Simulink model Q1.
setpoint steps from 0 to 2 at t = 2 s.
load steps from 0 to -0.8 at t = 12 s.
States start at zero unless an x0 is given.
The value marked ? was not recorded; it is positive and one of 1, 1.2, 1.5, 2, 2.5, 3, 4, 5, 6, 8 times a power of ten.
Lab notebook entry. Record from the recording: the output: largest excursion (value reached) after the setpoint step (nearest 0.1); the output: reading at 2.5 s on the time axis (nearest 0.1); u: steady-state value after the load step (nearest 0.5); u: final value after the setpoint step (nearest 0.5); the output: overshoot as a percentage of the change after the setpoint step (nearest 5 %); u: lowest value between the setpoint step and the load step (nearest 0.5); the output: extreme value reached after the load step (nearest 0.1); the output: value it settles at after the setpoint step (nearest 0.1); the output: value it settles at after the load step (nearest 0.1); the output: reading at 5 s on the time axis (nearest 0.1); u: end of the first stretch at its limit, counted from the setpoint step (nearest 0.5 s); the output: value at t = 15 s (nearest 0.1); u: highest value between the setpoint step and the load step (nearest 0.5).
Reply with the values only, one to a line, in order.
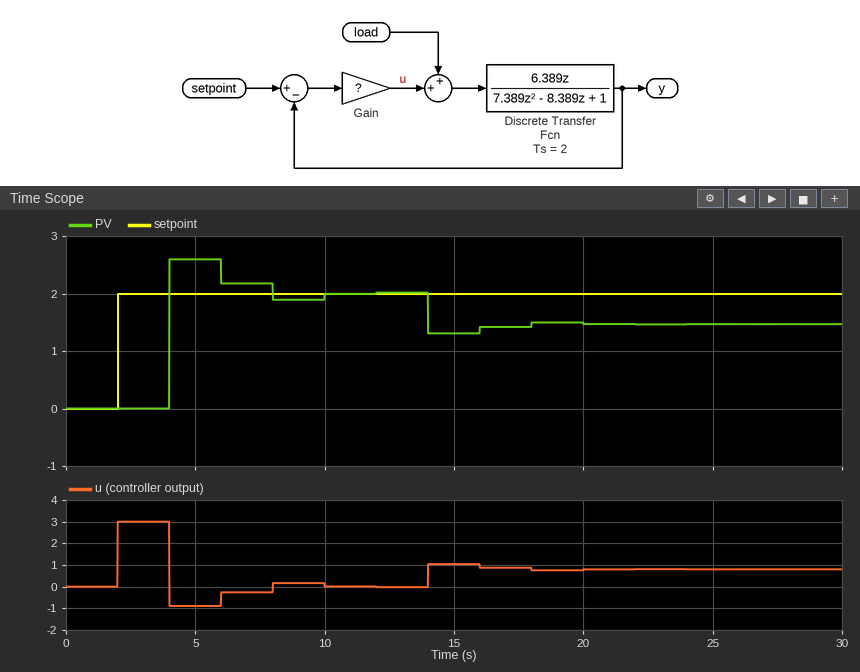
2.6
0.0
1.0
0.0
30 %
-1.0
1.3
2.0
1.5
2.6
2.0 s
1.3
3.0
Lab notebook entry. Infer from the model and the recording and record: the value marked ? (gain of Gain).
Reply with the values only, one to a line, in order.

1.5
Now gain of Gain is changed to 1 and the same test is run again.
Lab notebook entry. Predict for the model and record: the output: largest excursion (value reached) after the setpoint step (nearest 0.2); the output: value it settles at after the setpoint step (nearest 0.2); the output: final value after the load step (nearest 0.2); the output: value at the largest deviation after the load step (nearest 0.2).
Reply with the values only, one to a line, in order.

2.2
2.0
1.2
1.2
